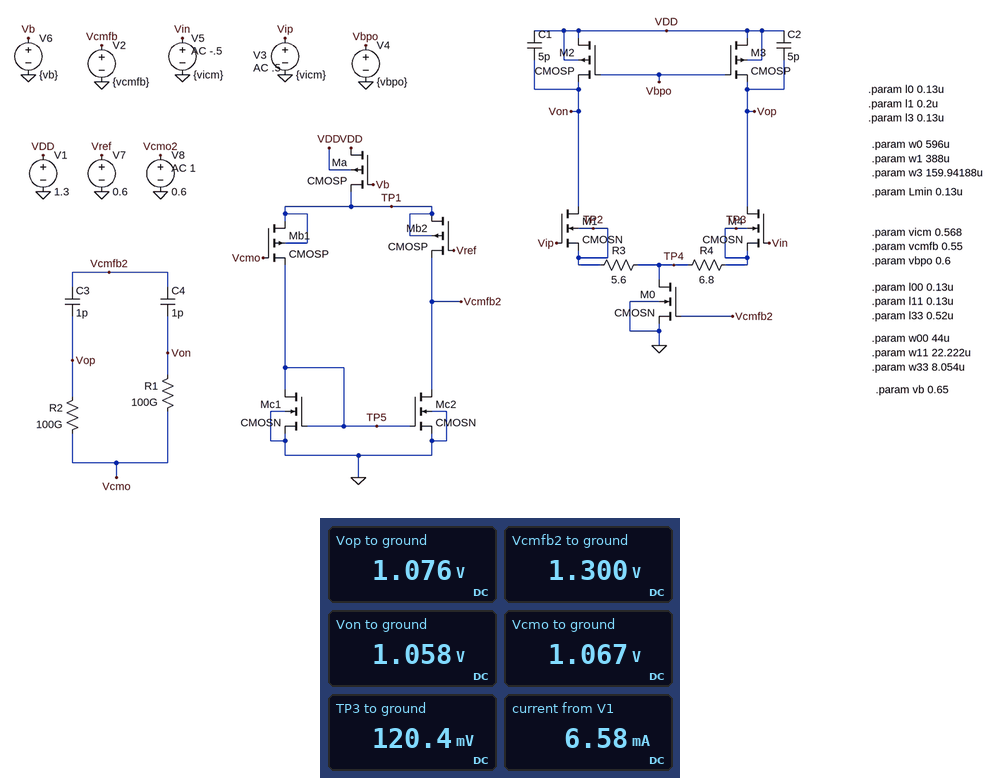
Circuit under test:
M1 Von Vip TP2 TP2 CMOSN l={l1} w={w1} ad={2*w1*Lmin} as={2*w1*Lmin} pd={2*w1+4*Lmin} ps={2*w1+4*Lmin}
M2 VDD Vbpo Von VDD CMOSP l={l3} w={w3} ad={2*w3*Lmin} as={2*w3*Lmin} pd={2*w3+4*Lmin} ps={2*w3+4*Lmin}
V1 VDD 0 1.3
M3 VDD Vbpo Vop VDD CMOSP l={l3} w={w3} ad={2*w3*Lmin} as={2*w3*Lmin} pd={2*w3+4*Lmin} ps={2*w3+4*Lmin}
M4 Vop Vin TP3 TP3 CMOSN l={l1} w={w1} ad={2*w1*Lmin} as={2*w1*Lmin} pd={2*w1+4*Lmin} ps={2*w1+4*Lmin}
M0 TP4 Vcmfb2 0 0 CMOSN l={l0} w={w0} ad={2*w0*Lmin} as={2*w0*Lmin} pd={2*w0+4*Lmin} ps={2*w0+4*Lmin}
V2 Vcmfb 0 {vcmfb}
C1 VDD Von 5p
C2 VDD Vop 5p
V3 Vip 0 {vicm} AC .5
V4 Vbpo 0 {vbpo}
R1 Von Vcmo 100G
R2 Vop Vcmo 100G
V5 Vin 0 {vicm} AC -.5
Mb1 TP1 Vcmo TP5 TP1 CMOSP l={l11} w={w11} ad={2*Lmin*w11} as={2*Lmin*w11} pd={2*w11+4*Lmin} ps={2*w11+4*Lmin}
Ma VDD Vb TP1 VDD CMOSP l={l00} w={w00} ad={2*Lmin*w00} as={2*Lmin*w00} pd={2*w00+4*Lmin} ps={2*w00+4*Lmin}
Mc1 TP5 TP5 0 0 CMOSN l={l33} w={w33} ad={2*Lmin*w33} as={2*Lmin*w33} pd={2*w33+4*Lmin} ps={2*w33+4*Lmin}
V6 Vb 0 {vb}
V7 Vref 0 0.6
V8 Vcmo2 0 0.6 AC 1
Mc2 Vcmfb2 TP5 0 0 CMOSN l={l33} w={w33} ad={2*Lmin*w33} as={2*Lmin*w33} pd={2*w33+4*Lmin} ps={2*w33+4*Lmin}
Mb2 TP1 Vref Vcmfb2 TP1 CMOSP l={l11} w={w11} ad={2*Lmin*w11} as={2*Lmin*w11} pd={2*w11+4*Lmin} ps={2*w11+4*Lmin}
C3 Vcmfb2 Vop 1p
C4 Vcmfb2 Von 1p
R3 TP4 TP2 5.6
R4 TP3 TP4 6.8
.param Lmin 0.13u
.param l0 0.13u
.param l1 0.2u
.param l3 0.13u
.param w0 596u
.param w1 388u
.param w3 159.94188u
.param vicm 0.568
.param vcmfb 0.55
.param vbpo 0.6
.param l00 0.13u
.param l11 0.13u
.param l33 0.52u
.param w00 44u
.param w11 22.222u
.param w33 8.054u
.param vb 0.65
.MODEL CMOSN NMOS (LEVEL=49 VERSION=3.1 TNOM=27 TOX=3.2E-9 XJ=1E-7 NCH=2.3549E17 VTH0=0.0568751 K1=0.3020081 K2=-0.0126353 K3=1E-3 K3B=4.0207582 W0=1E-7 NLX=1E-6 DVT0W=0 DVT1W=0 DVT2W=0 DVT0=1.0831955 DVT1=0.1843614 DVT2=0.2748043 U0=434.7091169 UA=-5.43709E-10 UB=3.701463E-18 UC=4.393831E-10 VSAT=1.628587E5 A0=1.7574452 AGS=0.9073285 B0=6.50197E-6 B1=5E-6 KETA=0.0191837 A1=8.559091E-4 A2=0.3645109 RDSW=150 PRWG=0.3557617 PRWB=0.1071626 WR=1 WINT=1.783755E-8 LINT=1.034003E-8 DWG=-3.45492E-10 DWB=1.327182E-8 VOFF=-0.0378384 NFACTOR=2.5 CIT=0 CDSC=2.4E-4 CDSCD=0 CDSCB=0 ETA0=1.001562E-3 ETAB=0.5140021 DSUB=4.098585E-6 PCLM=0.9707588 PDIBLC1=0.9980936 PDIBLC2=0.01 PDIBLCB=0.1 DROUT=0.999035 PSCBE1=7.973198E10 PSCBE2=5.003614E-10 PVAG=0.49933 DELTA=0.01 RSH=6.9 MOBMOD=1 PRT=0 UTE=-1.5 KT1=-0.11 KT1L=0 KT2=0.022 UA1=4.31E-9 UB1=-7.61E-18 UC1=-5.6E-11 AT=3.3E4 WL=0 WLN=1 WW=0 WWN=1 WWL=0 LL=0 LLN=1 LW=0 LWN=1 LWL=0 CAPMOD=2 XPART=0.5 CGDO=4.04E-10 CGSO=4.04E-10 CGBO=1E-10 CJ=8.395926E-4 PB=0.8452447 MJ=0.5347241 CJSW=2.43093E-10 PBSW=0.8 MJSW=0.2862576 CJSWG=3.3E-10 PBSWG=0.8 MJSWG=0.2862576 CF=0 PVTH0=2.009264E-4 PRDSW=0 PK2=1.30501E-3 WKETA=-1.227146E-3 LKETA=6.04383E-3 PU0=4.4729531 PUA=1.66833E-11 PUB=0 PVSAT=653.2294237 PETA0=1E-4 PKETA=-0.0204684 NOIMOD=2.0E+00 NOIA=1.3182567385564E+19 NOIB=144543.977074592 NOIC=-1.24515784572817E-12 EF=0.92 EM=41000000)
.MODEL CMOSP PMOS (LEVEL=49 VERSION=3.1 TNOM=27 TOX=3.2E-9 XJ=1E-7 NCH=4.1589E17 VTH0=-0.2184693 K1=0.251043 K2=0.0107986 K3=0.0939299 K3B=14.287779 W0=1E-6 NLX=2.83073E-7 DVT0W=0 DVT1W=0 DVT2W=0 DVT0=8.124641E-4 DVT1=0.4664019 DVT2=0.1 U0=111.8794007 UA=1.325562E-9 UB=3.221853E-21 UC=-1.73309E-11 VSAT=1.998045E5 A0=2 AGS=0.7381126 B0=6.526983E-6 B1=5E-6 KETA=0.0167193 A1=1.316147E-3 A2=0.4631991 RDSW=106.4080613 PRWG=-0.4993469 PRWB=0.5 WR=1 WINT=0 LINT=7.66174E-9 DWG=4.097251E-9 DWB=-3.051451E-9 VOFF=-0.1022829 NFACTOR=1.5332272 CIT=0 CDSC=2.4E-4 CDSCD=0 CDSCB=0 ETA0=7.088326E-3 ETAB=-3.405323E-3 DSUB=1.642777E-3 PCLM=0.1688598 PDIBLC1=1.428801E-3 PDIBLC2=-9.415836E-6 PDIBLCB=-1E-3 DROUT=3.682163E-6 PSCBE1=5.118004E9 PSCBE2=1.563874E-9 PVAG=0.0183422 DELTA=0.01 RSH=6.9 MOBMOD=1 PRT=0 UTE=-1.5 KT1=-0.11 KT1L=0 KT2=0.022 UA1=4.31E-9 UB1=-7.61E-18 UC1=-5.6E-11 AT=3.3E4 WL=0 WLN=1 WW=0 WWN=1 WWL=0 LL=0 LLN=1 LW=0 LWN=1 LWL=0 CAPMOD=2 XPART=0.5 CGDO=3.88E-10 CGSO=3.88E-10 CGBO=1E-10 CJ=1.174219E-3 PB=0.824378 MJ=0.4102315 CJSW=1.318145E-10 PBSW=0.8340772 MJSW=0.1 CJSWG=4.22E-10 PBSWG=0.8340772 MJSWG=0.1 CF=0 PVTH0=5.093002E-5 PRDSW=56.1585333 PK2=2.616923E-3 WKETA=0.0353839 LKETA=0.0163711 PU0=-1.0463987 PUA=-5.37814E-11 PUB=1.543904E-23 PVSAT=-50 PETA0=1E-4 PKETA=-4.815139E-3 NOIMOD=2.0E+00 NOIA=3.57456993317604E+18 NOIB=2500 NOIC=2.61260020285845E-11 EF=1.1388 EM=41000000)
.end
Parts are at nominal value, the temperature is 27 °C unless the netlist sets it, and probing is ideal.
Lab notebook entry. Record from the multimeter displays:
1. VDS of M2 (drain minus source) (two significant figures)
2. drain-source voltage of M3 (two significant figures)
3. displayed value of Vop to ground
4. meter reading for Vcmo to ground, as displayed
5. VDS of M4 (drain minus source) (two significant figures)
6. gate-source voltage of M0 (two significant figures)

240 mV
220 mV
1.076 V
1.067 V
960 mV
1.3 V
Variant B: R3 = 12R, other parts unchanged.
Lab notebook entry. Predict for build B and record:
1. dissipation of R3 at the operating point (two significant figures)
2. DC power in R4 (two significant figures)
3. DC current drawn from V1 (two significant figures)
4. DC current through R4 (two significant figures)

100 µW
77 µW
6.3 mA
3.4 mA
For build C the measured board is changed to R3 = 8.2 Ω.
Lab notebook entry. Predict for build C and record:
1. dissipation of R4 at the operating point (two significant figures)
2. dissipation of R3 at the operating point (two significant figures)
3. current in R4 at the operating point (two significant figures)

74 µW
82 µW
3.3 mA
